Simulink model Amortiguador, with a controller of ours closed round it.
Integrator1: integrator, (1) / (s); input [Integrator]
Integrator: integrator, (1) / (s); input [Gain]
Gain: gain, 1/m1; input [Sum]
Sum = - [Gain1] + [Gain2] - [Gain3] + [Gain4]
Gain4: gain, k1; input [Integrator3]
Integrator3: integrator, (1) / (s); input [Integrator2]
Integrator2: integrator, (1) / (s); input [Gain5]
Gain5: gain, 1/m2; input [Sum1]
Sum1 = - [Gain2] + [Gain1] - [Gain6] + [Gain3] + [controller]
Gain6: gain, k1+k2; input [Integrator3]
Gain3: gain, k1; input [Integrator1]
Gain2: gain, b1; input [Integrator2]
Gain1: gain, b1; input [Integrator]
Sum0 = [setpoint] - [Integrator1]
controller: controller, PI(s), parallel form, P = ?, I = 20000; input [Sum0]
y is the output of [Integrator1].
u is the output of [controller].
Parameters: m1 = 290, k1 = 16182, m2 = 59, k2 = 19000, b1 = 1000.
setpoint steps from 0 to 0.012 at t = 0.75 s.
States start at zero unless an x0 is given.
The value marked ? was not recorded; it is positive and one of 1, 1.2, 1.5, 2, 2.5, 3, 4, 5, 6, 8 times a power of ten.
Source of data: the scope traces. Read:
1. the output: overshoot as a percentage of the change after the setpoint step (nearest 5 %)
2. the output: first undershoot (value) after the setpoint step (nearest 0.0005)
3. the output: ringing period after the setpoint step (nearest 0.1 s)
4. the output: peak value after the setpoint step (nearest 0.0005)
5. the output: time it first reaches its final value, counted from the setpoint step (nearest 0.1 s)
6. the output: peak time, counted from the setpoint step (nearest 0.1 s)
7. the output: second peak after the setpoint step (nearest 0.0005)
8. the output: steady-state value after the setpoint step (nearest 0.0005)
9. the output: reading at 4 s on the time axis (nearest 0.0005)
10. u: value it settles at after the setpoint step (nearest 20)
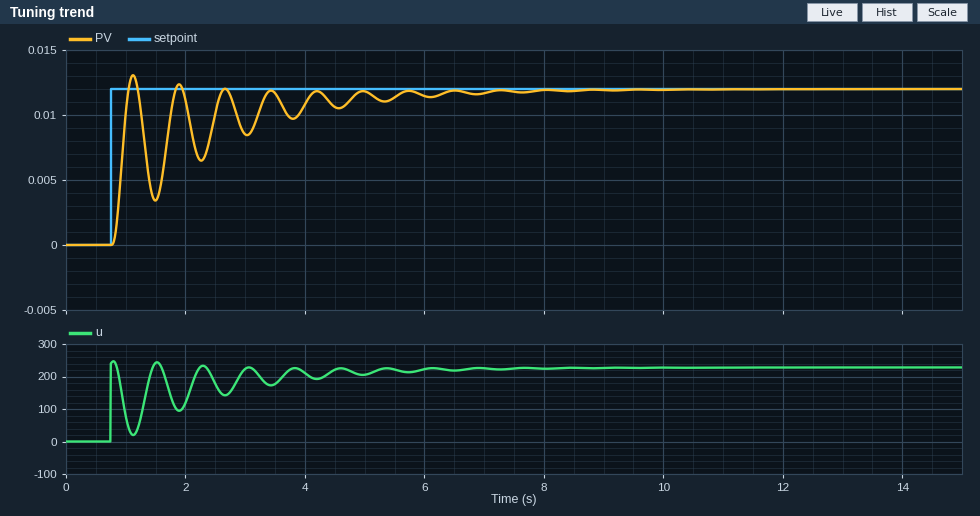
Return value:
10 %
0.0035
0.8 s
0.0130
0.3 s
0.4 s
0.0125
0.0120
0.0110
220
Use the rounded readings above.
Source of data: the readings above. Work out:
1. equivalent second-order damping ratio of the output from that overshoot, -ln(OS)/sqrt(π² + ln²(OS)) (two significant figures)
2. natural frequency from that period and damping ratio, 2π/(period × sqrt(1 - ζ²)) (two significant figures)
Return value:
0.59
9.7 rad/s
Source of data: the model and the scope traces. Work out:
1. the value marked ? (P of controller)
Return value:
20000
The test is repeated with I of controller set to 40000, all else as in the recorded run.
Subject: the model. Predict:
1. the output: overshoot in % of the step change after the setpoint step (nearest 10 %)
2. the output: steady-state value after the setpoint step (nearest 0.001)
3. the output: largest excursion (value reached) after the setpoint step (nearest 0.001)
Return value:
30 %
0.012
0.015
